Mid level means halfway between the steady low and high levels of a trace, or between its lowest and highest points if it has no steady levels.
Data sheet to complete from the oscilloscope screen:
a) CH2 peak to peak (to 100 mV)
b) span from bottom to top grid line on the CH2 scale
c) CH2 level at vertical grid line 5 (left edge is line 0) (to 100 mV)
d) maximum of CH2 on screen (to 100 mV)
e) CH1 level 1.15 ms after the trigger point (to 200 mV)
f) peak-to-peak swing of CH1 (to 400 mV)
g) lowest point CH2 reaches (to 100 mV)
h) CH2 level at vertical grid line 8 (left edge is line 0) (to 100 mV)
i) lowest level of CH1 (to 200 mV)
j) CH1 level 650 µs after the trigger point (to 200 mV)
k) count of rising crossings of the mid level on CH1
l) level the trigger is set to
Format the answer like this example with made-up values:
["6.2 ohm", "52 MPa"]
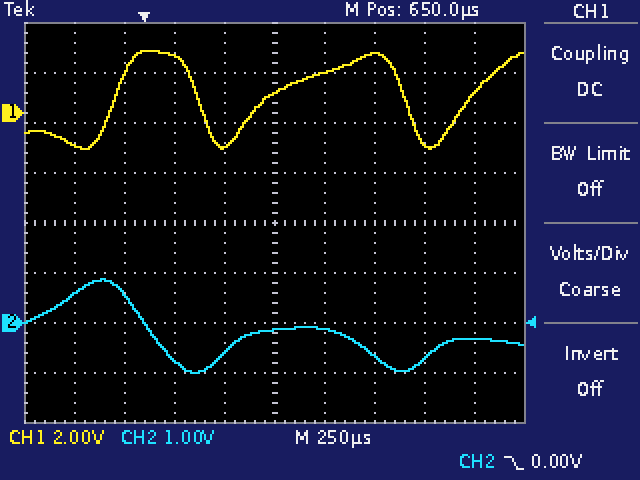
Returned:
["1.9 V", "8 V", "-100 mV", "900 mV", "2.4 V", "4.0 V", "-1.0 V", "-700 mV", "-1.4 V", "800 mV", "3", "0.00 V"]
